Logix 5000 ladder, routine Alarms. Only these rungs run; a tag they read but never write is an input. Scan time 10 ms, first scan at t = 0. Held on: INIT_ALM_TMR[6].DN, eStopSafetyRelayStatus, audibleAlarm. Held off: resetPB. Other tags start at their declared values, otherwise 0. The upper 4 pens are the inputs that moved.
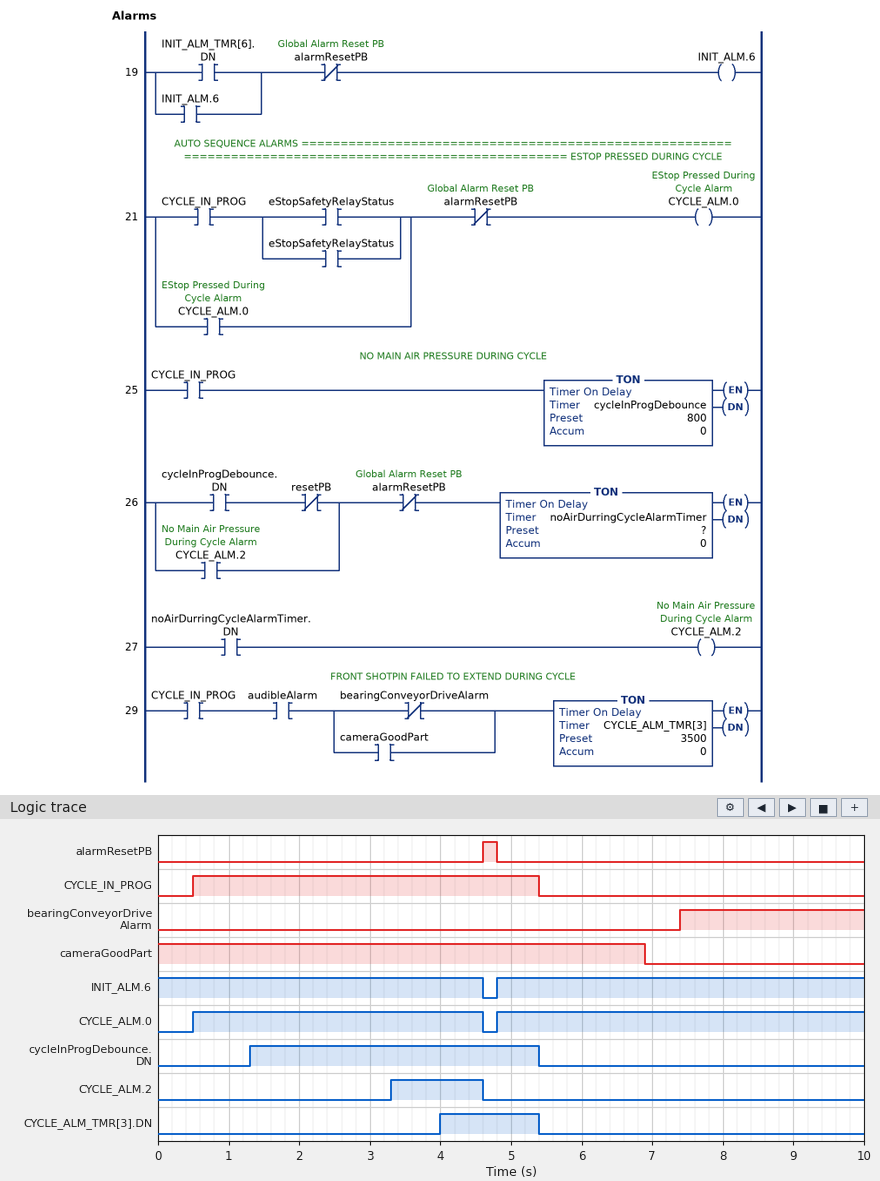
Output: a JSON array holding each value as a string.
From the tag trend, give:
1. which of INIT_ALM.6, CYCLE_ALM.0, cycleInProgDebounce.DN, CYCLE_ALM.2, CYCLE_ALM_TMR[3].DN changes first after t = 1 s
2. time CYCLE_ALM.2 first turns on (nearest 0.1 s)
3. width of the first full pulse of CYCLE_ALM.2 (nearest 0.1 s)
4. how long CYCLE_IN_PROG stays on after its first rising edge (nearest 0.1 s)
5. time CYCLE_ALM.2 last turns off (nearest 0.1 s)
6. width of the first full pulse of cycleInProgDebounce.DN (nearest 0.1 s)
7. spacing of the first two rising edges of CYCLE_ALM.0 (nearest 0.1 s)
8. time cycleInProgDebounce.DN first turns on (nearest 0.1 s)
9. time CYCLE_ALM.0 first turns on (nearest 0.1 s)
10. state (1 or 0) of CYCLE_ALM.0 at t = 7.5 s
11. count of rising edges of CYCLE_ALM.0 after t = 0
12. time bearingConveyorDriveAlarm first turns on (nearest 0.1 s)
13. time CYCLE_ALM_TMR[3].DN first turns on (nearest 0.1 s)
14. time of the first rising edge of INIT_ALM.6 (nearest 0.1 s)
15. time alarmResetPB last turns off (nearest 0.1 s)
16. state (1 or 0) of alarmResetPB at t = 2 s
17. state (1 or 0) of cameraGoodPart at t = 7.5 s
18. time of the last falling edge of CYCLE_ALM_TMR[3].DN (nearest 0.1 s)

["cycleInProgDebounce.DN", "3.3 s", "1.3 s", "4.9 s", "4.6 s", "4.1 s", "4.3 s", "1.3 s", "0.5 s", "1", "2", "7.4 s", "4.0 s", "4.8 s", "4.8 s", "0", "0", "5.4 s"]
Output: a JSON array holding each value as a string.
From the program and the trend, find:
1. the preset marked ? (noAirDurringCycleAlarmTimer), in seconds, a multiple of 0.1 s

["2.0 s"]
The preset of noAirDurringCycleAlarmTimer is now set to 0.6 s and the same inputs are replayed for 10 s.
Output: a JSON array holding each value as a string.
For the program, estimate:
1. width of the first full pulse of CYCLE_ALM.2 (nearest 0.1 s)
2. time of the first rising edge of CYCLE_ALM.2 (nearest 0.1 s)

["2.7 s", "1.9 s"]
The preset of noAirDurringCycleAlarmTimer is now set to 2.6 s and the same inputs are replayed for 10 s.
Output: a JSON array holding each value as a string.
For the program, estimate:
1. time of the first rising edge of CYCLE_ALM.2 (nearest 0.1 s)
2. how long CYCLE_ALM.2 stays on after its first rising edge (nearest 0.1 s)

["3.9 s", "0.7 s"]
